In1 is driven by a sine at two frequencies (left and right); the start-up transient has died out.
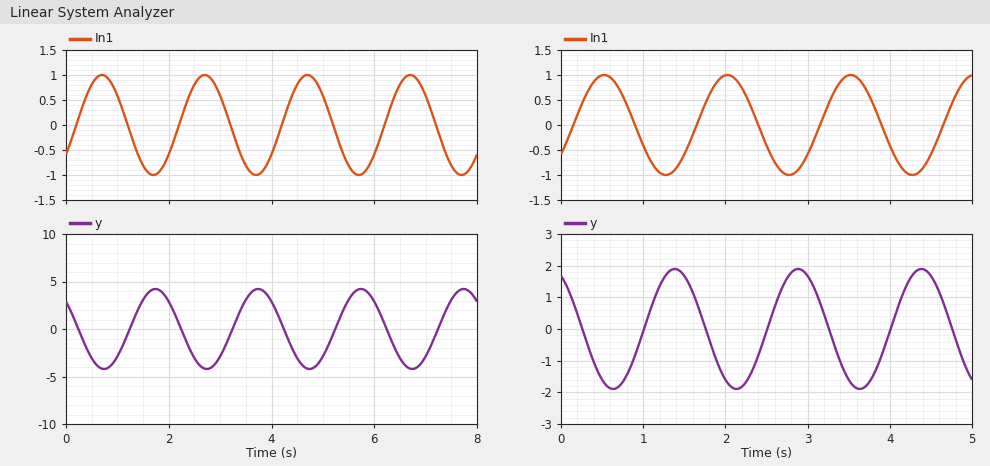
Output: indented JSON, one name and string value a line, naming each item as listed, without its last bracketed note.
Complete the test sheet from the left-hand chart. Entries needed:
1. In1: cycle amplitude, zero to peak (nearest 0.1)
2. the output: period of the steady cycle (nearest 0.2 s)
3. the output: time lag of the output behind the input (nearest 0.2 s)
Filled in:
{
  "In1: cycle amplitude, zero to peak": "1.0",
  "the output: period of the steady cycle": "2.0 s",
  "the output: time lag of the output behind the input": "1.0 s"
}
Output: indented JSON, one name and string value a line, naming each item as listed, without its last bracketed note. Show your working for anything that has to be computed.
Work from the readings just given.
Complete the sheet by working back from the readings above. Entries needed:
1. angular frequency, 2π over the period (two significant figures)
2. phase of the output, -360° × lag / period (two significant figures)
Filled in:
{
  "angular frequency, 2π over the period": "2π / 2 = 3.1 rad/s",
  "phase of the output, -360° × lag / period": "-360 × 1 / 2 = -180°"
}
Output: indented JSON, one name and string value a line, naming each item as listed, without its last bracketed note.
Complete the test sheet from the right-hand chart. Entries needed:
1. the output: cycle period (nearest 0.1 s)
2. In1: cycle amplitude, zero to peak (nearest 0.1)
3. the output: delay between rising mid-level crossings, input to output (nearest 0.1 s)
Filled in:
{
  "the output: cycle period": "1.5 s",
  "In1: cycle amplitude, zero to peak": "1.0",
  "the output: delay between rising mid-level crossings, input to output": "0.9 s"
}
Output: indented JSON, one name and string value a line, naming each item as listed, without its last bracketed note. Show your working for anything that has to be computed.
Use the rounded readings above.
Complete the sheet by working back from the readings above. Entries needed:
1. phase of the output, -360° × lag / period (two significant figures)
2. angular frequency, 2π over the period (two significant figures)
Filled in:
{
  "phase of the output, -360° × lag / period": "-360 × 0.9 / 1.5 = -220°",
  "angular frequency, 2π over the period": "2π / 1.5 = 4.2 rad/s"
}
